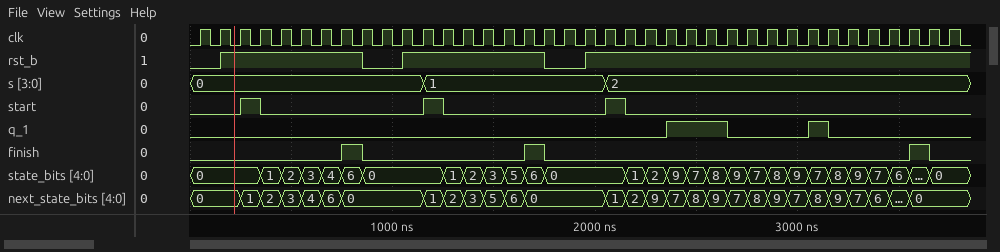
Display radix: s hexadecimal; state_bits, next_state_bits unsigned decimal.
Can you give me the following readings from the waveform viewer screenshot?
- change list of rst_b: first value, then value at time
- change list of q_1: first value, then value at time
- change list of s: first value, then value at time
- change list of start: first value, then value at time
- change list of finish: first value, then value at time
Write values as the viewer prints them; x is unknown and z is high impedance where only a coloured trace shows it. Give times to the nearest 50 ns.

0, 1 at 150 ns, 0 at 850 ns, 1 at 1050 ns, 0 at 1750 ns, 1 at 1950 ns
0, 1 at 2350 ns, 0 at 2650 ns, 1 at 3050 ns, 0 at 3150 ns
0, 1 at 1150 ns, 2 at 2050 ns
0, 1 at 250 ns, 0 at 350 ns, 1 at 1150 ns, 0 at 1250 ns, 1 at 2050 ns, 0 at 2150 ns
0, 1 at 750 ns, 0 at 850 ns, 1 at 1650 ns, 0 at 1750 ns, 1 at 3550 ns, 0 at 3650 ns
